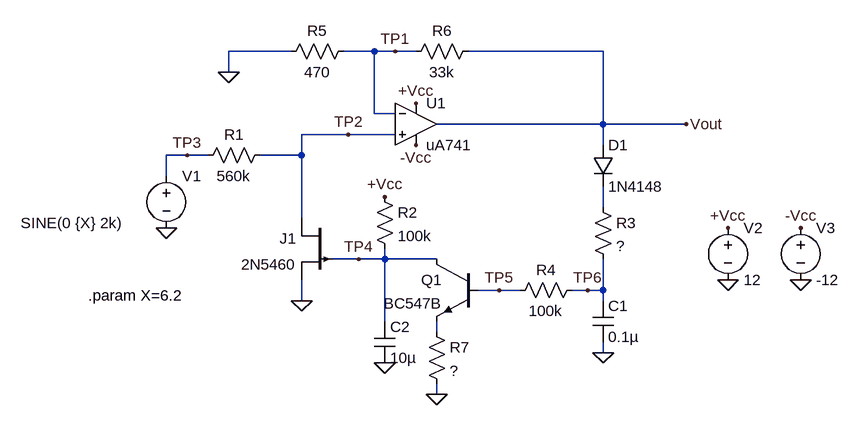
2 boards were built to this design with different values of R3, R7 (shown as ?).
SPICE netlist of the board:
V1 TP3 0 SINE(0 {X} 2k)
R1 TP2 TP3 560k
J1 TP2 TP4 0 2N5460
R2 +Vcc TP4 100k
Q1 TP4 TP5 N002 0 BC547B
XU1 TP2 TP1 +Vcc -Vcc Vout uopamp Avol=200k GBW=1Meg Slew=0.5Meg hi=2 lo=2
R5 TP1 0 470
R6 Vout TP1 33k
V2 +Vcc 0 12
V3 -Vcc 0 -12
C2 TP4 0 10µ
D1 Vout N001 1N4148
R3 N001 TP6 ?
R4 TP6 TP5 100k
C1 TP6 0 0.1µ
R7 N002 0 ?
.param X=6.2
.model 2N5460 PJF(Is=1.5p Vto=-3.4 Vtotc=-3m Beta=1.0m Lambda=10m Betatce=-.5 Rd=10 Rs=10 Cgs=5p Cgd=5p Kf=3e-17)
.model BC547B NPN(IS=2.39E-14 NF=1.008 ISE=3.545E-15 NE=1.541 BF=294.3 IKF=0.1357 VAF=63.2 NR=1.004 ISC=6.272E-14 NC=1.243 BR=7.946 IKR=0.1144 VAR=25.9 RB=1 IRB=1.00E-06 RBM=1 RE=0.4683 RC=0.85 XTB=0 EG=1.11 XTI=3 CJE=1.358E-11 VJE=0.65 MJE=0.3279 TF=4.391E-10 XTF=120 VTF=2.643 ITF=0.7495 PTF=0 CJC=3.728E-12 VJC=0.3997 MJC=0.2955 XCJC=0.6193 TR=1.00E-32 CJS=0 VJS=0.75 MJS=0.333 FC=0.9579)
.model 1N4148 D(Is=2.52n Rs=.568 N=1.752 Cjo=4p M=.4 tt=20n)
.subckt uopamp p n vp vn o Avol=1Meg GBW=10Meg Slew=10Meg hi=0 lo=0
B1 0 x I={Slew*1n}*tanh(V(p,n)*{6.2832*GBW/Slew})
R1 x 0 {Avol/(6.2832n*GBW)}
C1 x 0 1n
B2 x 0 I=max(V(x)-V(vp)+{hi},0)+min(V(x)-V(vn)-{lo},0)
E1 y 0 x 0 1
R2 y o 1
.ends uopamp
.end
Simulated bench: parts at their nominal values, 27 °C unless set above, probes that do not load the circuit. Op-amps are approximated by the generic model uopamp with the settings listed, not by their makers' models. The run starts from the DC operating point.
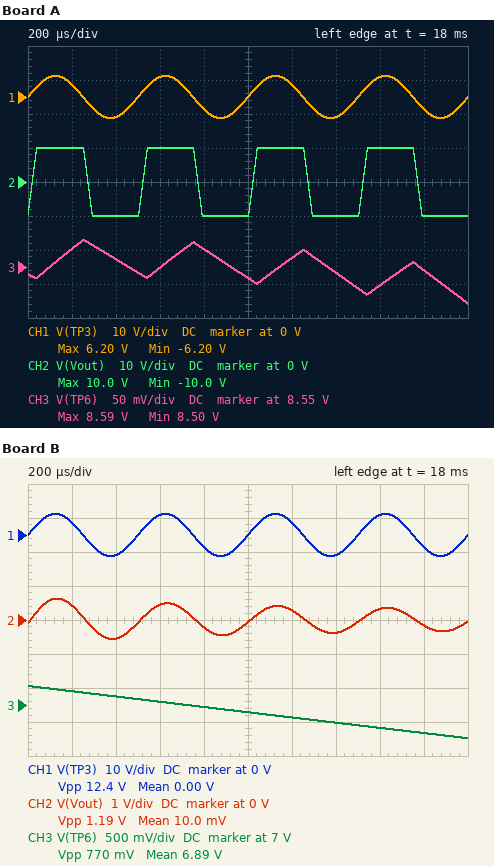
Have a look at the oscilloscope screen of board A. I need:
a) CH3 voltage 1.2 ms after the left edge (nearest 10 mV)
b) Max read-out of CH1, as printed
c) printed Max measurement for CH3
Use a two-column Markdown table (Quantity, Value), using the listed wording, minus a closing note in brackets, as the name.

| Quantity | Value |
|---|---|
| CH3 voltage 1.2 ms after the left edge | 8.56 V |
| Max read-out of CH1, as printed | 6.20 V |
| printed Max measurement for CH3 | 8.59 V |
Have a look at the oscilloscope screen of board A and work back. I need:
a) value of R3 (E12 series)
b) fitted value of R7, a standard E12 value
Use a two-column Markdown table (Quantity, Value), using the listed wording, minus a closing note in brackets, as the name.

| Quantity | Value |
|---|---|
| value of R3 | 22 kΩ |
| fitted value of R7, a standard E12 value | 1.5 kΩ |
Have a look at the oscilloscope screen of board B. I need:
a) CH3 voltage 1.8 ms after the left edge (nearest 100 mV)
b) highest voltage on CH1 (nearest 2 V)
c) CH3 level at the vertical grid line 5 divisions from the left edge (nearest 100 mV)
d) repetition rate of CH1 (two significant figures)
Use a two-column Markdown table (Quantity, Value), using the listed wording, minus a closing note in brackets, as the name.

| Quantity | Value |
|---|---|
| CH3 voltage 1.8 ms after the left edge | 6.6 V |
| highest voltage on CH1 | 6 V |
| CH3 level at the vertical grid line 5 divisions from the left edge | 6.9 V |
| repetition rate of CH1 | 2.0 kHz |
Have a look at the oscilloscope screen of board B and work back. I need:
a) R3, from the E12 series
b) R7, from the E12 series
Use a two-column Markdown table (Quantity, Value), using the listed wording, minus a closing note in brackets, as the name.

| Quantity | Value |
|---|---|
| R3, from the E12 series | 22 kΩ |
| R7, from the E12 series | 680 Ω |
